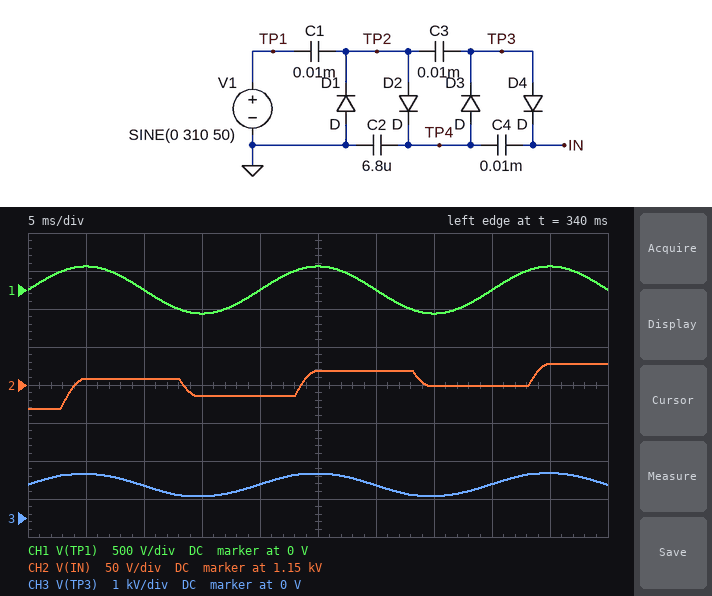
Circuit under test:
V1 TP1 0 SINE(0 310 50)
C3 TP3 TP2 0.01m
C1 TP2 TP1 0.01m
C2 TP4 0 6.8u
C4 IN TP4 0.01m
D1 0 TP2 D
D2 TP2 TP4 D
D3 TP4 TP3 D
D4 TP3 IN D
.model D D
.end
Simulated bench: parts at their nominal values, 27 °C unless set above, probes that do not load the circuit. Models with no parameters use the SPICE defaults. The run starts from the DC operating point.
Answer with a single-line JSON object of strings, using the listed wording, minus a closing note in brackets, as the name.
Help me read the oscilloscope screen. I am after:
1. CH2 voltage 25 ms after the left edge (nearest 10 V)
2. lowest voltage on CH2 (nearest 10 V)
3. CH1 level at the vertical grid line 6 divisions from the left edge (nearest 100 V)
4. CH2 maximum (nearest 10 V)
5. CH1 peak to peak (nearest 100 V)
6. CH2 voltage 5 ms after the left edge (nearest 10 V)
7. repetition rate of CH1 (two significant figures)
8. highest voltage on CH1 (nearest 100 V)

{"CH2 voltage 25 ms after the left edge": "1.17 kV", "lowest voltage on CH2": "1.12 kV", "CH1 level at the vertical grid line 6 divisions from the left edge": "0 V", "CH2 maximum": "1.18 kV", "CH1 peak to peak": "600 V", "CH2 voltage 5 ms after the left edge": "1.16 kV", "repetition rate of CH1": "50 Hz", "highest voltage on CH1": "300 V"}
